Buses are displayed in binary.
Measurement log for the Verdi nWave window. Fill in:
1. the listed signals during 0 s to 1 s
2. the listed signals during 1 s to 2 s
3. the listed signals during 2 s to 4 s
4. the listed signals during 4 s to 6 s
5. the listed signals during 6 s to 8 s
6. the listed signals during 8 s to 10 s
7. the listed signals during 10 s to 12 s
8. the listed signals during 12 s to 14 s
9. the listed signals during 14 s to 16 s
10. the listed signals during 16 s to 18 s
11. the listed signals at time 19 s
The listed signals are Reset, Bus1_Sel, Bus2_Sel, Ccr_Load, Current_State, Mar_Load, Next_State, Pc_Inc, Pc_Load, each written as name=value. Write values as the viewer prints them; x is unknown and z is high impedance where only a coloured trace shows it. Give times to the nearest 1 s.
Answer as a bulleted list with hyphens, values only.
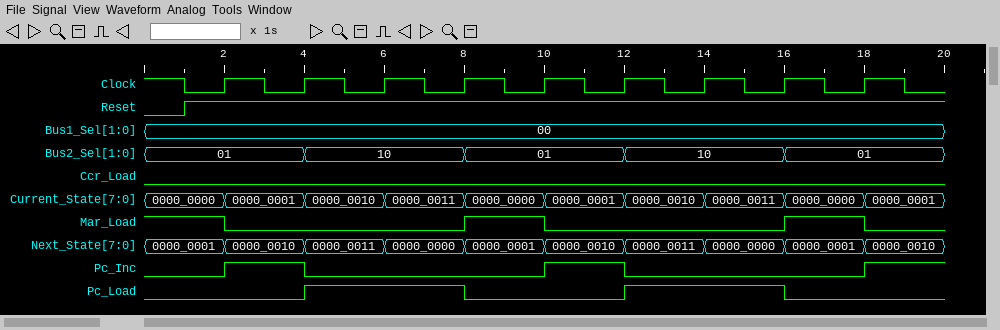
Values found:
- Reset=0, Bus1_Sel=00, Bus2_Sel=01, Ccr_Load=0, Current_State=0000_0000, Mar_Load=1, Next_State=0000_0001, Pc_Inc=0, Pc_Load=0
- Reset=1, Bus1_Sel=00, Bus2_Sel=01, Ccr_Load=0, Current_State=0000_0000, Mar_Load=1, Next_State=0000_0001, Pc_Inc=0, Pc_Load=0
- Reset=1, Bus1_Sel=00, Bus2_Sel=01, Ccr_Load=0, Current_State=0000_0001, Mar_Load=0, Next_State=0000_0010, Pc_Inc=1, Pc_Load=0
- Reset=1, Bus1_Sel=00, Bus2_Sel=10, Ccr_Load=0, Current_State=0000_0010, Mar_Load=0, Next_State=0000_0011, Pc_Inc=0, Pc_Load=1
- Reset=1, Bus1_Sel=00, Bus2_Sel=10, Ccr_Load=0, Current_State=0000_0011, Mar_Load=0, Next_State=0000_0000, Pc_Inc=0, Pc_Load=1
- Reset=1, Bus1_Sel=00, Bus2_Sel=01, Ccr_Load=0, Current_State=0000_0000, Mar_Load=1, Next_State=0000_0001, Pc_Inc=0, Pc_Load=0
- Reset=1, Bus1_Sel=00, Bus2_Sel=01, Ccr_Load=0, Current_State=0000_0001, Mar_Load=0, Next_State=0000_0010, Pc_Inc=1, Pc_Load=0
- Reset=1, Bus1_Sel=00, Bus2_Sel=10, Ccr_Load=0, Current_State=0000_0010, Mar_Load=0, Next_State=0000_0011, Pc_Inc=0, Pc_Load=1
- Reset=1, Bus1_Sel=00, Bus2_Sel=10, Ccr_Load=0, Current_State=0000_0011, Mar_Load=0, Next_State=0000_0000, Pc_Inc=0, Pc_Load=1
- Reset=1, Bus1_Sel=00, Bus2_Sel=01, Ccr_Load=0, Current_State=0000_0000, Mar_Load=1, Next_State=0000_0001, Pc_Inc=0, Pc_Load=0
- Reset=1, Bus1_Sel=00, Bus2_Sel=01, Ccr_Load=0, Current_State=0000_0001, Mar_Load=0, Next_State=0000_0010, Pc_Inc=1, Pc_Load=0
